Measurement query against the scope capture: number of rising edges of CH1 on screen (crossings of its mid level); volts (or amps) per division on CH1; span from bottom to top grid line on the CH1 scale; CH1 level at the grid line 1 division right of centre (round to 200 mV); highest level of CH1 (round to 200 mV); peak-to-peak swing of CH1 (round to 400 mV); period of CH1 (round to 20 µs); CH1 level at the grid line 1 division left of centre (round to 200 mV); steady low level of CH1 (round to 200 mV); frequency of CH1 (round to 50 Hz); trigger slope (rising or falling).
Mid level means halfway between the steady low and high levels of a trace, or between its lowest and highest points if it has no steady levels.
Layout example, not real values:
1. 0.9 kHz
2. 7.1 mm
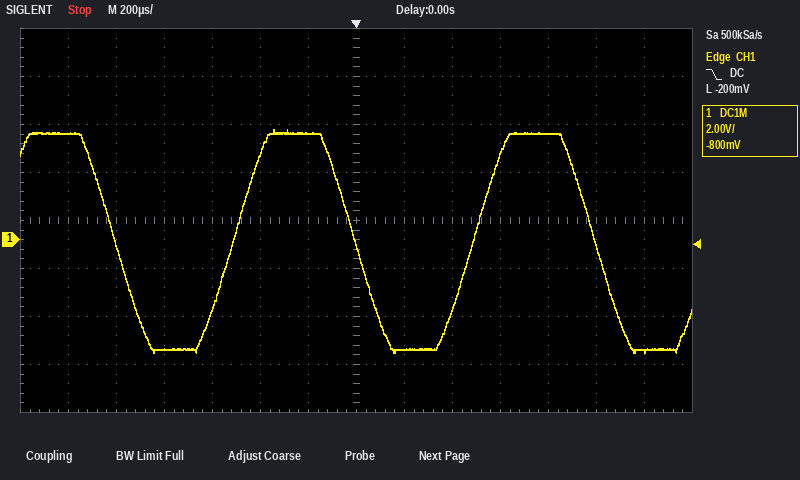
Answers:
1. 2
2. 2 V
3. 16 V
4. -4.6 V
5. 4.6 V
6. 9.2 V
7. 1.00 ms
8. 4.4 V
9. -4.6 V
10. 1.00 kHz
11. falling
